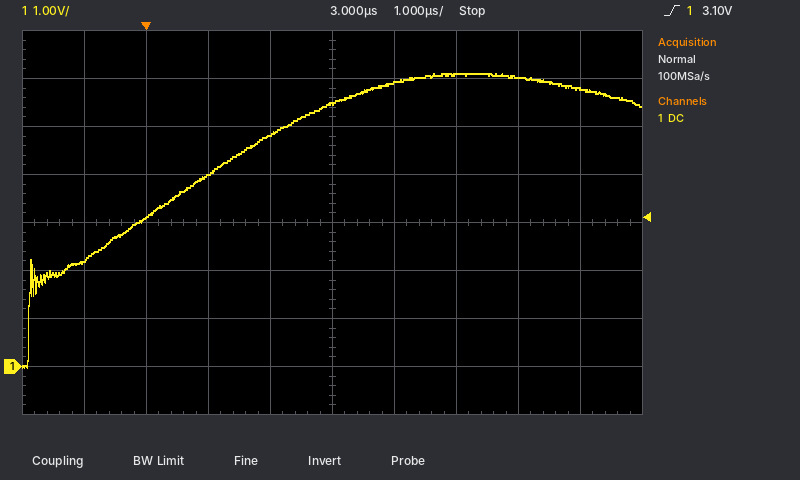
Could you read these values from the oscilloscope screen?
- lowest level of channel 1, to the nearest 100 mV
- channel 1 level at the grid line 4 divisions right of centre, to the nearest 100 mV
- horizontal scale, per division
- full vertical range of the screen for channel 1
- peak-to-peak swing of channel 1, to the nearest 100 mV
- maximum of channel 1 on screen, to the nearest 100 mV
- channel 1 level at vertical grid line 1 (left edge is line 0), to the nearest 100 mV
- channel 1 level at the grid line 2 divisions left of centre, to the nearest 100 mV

0.0 V
5.8 V
1 µs
8 V
6.1 V
6.1 V
2.2 V
4.0 V
